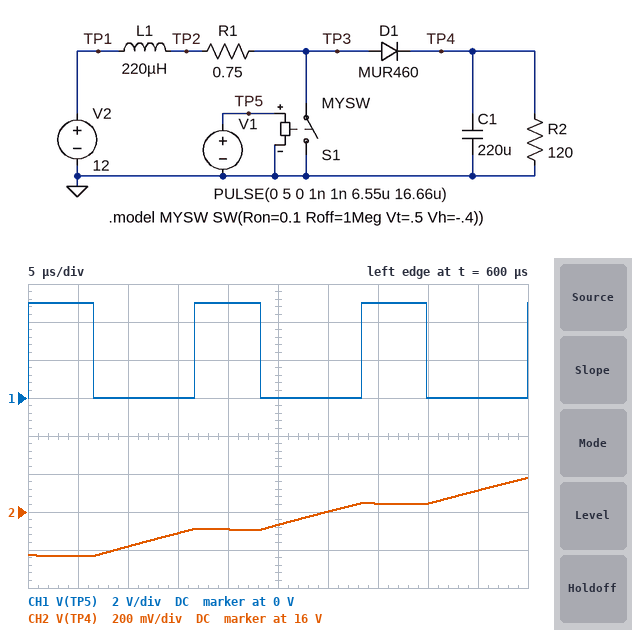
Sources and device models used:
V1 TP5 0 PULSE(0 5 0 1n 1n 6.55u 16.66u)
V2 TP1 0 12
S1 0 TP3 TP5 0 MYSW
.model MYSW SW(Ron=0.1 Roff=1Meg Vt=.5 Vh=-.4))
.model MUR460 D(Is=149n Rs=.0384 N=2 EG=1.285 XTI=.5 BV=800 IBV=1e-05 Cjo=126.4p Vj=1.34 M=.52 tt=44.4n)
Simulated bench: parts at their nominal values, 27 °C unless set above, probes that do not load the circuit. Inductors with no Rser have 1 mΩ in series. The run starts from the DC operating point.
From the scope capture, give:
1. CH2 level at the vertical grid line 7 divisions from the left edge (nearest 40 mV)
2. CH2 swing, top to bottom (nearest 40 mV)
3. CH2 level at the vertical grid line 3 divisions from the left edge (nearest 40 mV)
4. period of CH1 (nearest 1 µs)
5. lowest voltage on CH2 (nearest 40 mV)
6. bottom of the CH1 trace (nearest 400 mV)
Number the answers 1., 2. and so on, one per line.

1. 16.04 V
2. 400 mV
3. 15.88 V
4. 17 µs
5. 15.76 V
6. 0 V
